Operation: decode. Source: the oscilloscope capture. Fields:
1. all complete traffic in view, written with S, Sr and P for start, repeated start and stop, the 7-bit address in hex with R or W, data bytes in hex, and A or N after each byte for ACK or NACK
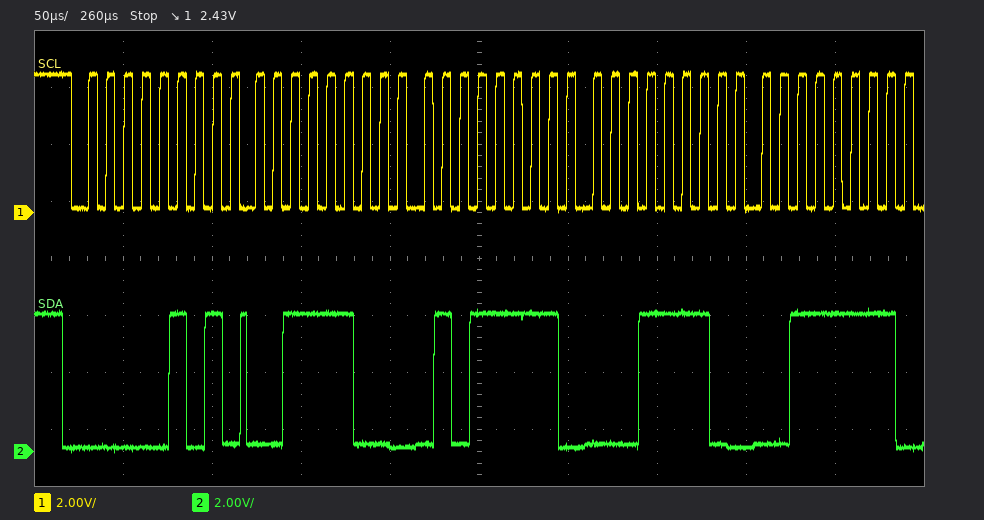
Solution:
S 02R A 3C A 5F A 1E A 3F A
